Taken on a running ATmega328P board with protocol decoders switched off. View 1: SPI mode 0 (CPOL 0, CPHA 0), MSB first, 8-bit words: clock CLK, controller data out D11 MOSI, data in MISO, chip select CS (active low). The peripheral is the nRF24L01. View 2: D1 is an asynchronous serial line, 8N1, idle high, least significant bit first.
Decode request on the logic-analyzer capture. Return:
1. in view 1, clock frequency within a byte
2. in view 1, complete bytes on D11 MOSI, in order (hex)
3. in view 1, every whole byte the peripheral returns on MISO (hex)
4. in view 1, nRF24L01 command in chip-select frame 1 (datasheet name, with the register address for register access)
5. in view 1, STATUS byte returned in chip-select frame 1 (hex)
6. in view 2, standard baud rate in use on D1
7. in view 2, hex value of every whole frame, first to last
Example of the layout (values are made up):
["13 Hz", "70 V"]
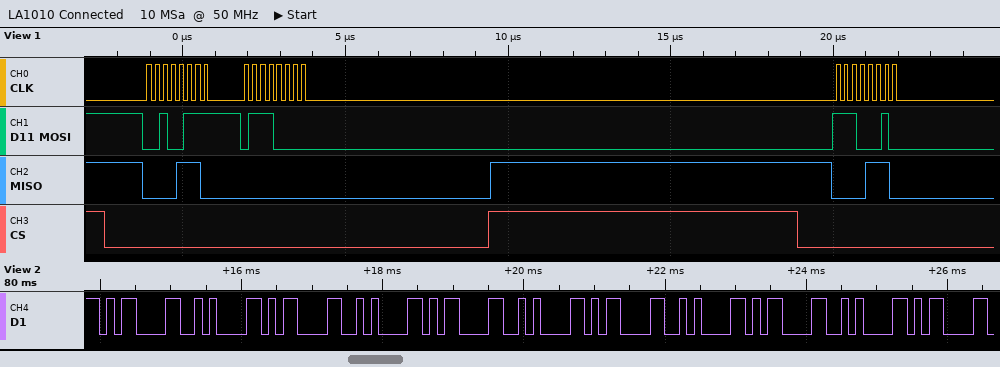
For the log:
["4 MHz", "27 70 E2", "0E 00 0E", "W_REGISTER 0x07", "0x0E", "9600 baud", "0D 0A 0D 0A 0D 0A 0D 0A 0D 0A 0D"]
